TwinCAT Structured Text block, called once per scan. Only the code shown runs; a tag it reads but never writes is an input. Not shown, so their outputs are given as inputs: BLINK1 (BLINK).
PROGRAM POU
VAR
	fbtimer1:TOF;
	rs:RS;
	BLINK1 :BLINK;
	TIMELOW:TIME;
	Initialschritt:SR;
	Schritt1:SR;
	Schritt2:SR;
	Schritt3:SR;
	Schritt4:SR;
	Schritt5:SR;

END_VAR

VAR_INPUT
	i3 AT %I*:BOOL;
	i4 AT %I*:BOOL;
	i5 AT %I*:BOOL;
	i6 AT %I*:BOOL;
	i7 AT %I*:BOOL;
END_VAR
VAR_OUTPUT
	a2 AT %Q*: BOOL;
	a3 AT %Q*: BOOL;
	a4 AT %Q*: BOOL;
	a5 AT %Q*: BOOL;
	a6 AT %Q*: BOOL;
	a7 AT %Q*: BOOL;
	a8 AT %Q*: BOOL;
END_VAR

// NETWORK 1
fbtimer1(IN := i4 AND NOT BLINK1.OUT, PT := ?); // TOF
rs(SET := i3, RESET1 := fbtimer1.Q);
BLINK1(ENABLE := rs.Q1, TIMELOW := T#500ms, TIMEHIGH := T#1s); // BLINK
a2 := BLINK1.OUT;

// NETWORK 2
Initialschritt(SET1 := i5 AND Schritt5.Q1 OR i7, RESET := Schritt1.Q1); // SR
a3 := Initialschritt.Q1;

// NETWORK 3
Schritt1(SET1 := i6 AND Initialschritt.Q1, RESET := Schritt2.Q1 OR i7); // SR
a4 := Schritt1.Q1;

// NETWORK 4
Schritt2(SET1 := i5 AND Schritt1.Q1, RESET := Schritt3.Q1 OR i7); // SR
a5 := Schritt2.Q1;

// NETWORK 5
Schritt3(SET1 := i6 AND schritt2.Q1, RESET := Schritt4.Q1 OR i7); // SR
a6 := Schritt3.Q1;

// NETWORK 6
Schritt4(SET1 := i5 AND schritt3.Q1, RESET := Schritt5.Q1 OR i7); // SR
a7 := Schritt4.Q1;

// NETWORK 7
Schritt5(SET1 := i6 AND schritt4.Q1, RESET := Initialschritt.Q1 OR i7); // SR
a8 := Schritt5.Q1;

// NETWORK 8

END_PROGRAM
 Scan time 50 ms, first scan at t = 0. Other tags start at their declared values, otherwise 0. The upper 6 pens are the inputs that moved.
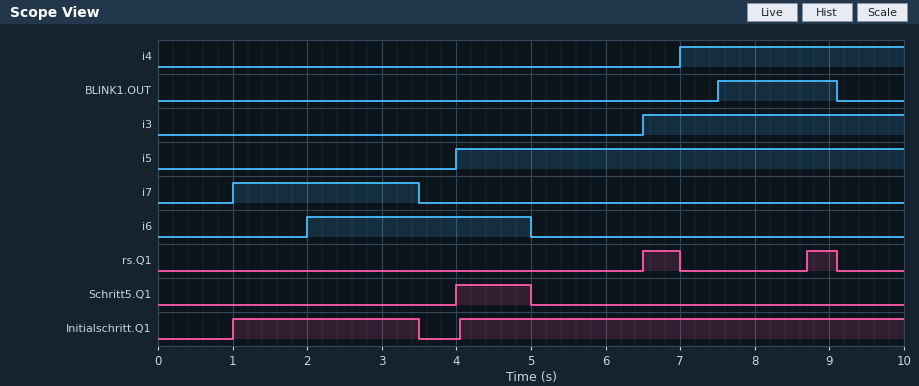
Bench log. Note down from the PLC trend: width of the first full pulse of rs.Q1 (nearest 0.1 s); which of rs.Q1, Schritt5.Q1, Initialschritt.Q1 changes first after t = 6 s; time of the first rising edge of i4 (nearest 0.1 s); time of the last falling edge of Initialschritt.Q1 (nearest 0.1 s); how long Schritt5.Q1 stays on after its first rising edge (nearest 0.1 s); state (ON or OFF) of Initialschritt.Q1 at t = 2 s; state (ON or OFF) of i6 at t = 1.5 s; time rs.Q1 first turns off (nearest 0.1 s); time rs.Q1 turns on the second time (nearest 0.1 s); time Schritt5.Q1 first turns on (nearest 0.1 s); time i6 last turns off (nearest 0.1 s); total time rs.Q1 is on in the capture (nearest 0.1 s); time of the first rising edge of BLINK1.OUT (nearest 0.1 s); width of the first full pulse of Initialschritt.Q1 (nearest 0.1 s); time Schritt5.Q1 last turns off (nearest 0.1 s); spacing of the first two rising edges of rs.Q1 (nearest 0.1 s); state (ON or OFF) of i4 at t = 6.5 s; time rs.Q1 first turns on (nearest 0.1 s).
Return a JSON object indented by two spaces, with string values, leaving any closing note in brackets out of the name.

{
  "width of the first full pulse of rs.Q1": "0.5 s",
  "which of rs.Q1, Schritt5.Q1, Initialschritt.Q1 changes first after t = 6 s": "rs.Q1",
  "time of the first rising edge of i4": "7.0 s",
  "time of the last falling edge of Initialschritt.Q1": "3.5 s",
  "how long Schritt5.Q1 stays on after its first rising edge": "1.0 s",
  "state (ON or OFF) of Initialschritt.Q1 at t = 2 s": "ON",
  "state (ON or OFF) of i6 at t = 1.5 s": "OFF",
  "time rs.Q1 first turns off": "7.0 s",
  "time rs.Q1 turns on the second time": "8.7 s",
  "time Schritt5.Q1 first turns on": "4.0 s",
  "time i6 last turns off": "5.0 s",
  "total time rs.Q1 is on in the capture": "0.9 s",
  "time of the first rising edge of BLINK1.OUT": "7.5 s",
  "width of the first full pulse of Initialschritt.Q1": "2.5 s",
  "time Schritt5.Q1 last turns off": "5.0 s",
  "spacing of the first two rising edges of rs.Q1": "2.2 s",
  "state (ON or OFF) of i4 at t = 6.5 s": "OFF",
  "time rs.Q1 first turns on": "6.5 s"
}
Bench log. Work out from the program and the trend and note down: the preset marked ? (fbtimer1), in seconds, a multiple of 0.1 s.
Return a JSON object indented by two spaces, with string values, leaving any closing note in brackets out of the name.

{
  "the preset marked ? (fbtimer1), in seconds, a multiple of 0.1 s": "1.2 s"
}
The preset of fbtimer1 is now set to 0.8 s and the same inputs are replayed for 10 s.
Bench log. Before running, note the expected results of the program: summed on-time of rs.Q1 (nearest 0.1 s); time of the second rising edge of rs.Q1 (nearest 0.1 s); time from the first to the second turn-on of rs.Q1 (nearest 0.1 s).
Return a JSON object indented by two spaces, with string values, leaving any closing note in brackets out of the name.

{
  "summed on-time of rs.Q1": "1.3 s",
  "time of the second rising edge of rs.Q1": "8.3 s",
  "time from the first to the second turn-on of rs.Q1": "1.8 s"
}
